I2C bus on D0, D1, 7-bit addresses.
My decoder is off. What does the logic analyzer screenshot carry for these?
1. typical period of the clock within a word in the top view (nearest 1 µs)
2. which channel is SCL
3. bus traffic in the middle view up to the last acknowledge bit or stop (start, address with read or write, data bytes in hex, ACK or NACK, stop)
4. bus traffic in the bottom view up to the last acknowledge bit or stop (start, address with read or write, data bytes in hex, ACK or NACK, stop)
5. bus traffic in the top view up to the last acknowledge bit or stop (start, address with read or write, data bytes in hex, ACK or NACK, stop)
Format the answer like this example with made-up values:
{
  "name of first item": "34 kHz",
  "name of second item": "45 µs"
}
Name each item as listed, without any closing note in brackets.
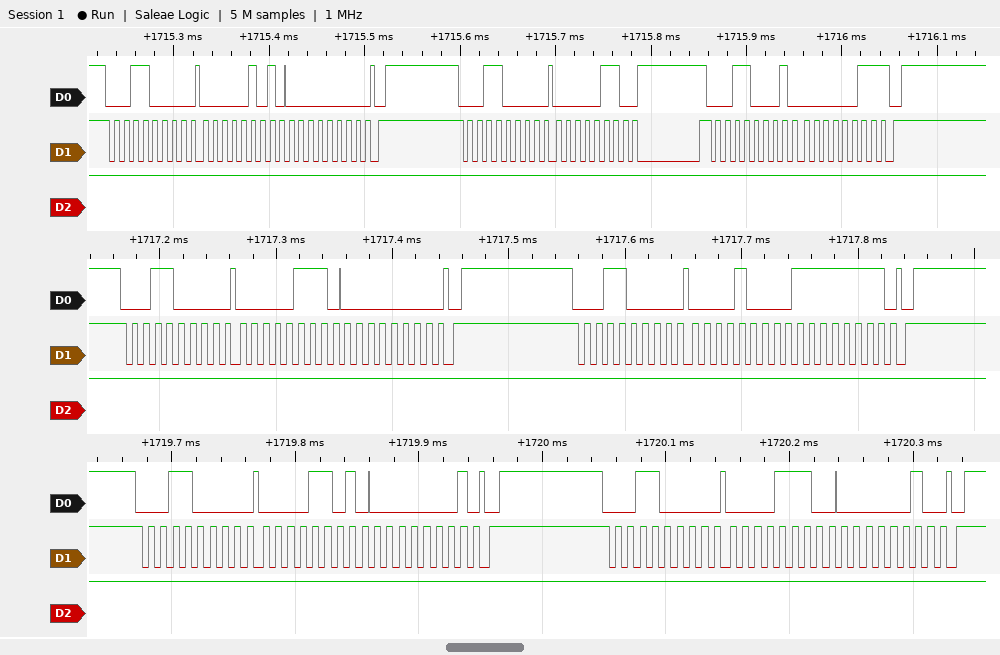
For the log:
{
  "typical period of the clock within a word in the top view": "10 µs",
  "which channel is SCL": "D1",
  "bus traffic in the middle view up to the last acknowledge bit or stop": "start, address 18 write ACK, 07 ACK, 00 ACK, stop, start, address 18 write ACK, 08 ACK, FF ACK, stop",
  "bus traffic in the bottom view up to the last acknowledge bit or stop": "start, address 18 write ACK, 0D ACK, 01 ACK, stop, start, address 18 write ACK, 0E ACK, 02 ACK, stop",
  "bus traffic in the top view up to the last acknowledge bit or stop": "start, address 18 write ACK, 05 ACK, 00 ACK, stop, start, address 18 write ACK, 06 ACK, repeated start, address 18 read ACK, 03 NACK, stop"
}
